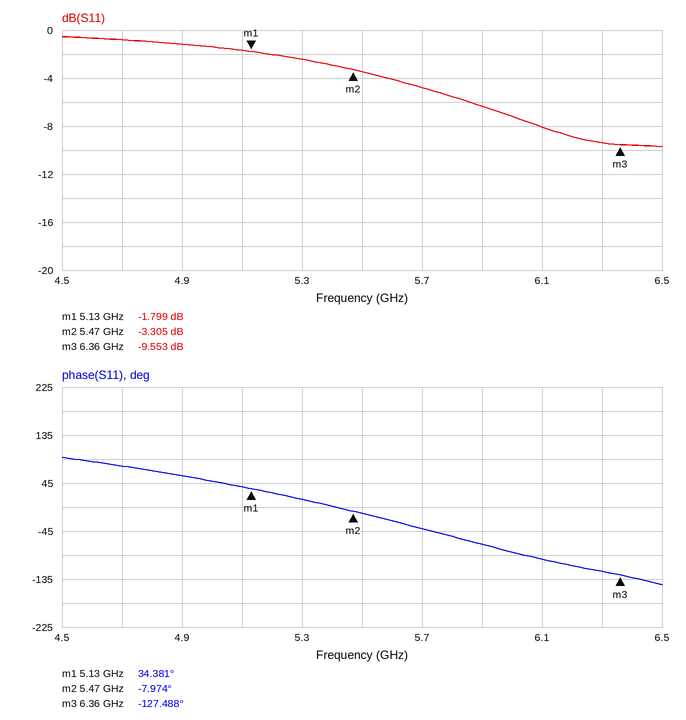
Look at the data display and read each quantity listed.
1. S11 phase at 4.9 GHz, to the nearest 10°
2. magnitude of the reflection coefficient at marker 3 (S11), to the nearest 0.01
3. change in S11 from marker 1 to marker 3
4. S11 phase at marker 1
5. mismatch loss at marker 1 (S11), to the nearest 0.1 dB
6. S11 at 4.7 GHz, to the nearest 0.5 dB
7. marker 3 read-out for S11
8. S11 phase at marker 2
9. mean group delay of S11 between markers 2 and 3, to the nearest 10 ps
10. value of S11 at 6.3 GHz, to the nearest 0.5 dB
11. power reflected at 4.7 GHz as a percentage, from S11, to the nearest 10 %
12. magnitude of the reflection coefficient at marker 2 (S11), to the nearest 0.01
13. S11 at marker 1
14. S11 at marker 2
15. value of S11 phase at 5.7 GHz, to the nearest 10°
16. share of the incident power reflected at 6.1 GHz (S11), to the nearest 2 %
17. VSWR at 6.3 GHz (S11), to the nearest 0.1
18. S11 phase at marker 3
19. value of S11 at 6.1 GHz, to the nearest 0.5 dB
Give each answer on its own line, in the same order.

60°
0.33
-7.754 dB
34.381°
4.7 dB
-1.0 dB
-9.553 dB
-7.974°
370 ps
-9.5 dB
80 %
0.68
-1.799 dB
-3.305 dB
-40°
16 %
2.0
-127.488°
-8.0 dB
